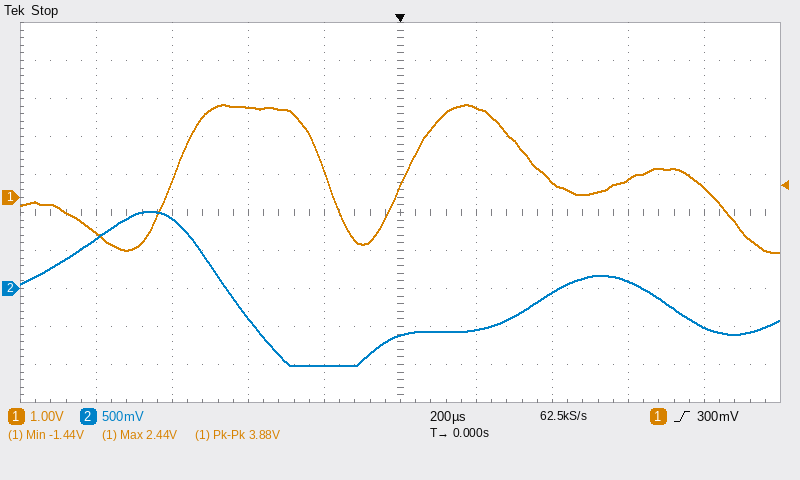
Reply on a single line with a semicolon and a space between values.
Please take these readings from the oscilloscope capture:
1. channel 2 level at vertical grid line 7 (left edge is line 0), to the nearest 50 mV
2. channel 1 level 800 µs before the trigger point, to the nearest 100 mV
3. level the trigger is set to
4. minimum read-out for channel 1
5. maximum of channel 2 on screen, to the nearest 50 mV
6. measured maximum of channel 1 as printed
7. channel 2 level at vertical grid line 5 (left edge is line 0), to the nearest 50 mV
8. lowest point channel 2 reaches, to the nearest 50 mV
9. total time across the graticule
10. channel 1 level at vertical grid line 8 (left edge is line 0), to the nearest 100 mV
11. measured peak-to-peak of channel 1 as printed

-50 mV; -900 mV; 300 mV; -1.44 V; 1.00 V; 2.44 V; -600 mV; -1.00 V; 2 ms; 500 mV; 3.88 V
